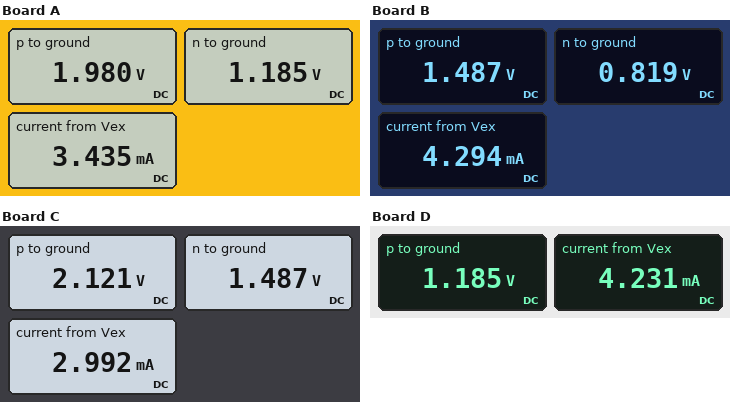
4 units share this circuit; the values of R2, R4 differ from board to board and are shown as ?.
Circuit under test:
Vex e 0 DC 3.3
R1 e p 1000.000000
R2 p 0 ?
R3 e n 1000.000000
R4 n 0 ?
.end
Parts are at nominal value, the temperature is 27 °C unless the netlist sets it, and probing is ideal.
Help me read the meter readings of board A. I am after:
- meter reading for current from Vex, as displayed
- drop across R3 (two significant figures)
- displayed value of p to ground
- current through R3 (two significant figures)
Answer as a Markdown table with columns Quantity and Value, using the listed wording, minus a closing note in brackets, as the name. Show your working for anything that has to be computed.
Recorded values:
| Quantity | Value |
|---|---|
| meter reading for current from Vex, as displayed | 3.435 mA |
| drop across R3 | 3.3 V - 1.185 V = 2.1 V |
| displayed value of p to ground | 1.980 V |
| current through R3 | (3.3 V - 1.185 V) / 1 kΩ = 2.1 mA |
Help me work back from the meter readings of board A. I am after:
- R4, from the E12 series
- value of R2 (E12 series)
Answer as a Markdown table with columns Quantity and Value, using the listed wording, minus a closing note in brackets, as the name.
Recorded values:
| Quantity | Value |
|---|---|
| R4, from the E12 series | 560 Ω |
| value of R2 | 1.5 kΩ |
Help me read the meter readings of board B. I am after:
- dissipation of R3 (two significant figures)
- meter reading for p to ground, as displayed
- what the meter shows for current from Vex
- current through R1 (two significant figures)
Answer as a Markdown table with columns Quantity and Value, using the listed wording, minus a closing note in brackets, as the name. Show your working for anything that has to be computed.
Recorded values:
| Quantity | Value |
|---|---|
| dissipation of R3 | (3.3 V - 819 mV)^2 / 1 kΩ = 6.2 mW |
| meter reading for p to ground, as displayed | 1.487 V |
| what the meter shows for current from Vex | 4.294 mA |
| current through R1 | (3.3 V - 1.487 V) / 1 kΩ = 1.8 mA |
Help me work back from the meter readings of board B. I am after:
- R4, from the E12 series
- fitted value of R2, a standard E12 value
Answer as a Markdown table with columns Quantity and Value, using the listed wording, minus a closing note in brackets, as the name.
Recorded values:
| Quantity | Value |
|---|---|
| R4, from the E12 series | 330 Ω |
| fitted value of R2, a standard E12 value | 820 Ω |
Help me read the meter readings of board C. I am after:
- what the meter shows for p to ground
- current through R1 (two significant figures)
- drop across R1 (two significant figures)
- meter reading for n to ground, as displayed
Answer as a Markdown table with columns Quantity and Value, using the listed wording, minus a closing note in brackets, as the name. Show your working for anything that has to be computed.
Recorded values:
| Quantity | Value |
|---|---|
| what the meter shows for p to ground | 2.121 V |
| current through R1 | (3.3 V - 2.121 V) / 1 kΩ = 1.2 mA |
| drop across R1 | 3.3 V - 2.121 V = 1.2 V |
| meter reading for n to ground, as displayed | 1.487 V |
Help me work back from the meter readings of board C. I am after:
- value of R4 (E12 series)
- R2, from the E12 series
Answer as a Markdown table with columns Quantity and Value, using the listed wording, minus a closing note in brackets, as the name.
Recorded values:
| Quantity | Value |
|---|---|
| value of R4 | 820 Ω |
| R2, from the E12 series | 1.8 kΩ |
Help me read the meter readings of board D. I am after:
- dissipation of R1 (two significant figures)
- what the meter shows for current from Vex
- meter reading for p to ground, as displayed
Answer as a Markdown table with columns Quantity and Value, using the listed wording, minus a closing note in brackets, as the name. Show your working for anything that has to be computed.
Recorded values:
| Quantity | Value |
|---|---|
| dissipation of R1 | (3.3 V - 1.185 V)^2 / 1 kΩ = 4.5 mW |
| what the meter shows for current from Vex | 4.231 mA |
| meter reading for p to ground, as displayed | 1.185 V |
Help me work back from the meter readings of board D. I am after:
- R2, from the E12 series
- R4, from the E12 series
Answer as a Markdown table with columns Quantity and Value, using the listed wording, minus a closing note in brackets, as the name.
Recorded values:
| Quantity | Value |
|---|---|
| R2, from the E12 series | 560 Ω |
| R4, from the E12 series | 560 Ω |
